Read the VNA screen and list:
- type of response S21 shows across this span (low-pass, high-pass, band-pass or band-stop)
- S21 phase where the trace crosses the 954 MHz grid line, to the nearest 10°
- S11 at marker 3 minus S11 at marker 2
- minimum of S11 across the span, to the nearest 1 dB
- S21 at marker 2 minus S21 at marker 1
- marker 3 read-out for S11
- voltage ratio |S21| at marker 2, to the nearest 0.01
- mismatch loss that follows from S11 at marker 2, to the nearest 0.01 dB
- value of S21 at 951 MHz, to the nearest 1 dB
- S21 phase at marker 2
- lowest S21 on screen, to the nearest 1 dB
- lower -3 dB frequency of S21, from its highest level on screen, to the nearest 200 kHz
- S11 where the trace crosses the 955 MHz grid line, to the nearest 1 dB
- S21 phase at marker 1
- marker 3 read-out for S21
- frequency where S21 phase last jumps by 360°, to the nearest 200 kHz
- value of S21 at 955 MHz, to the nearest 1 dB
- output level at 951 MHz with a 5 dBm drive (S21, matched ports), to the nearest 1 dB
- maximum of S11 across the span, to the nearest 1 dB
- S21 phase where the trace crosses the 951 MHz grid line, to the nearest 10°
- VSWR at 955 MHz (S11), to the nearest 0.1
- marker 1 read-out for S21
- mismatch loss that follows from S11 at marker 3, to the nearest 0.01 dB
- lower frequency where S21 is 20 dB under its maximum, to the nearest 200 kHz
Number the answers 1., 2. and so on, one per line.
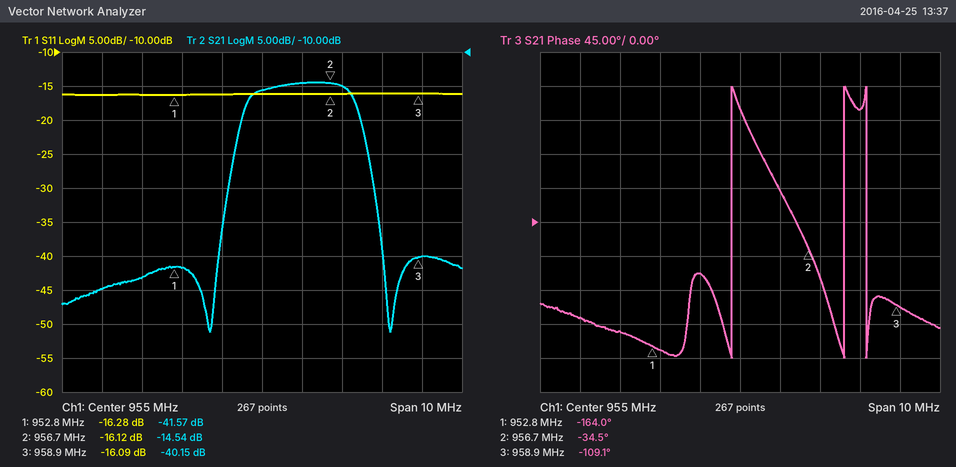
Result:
1. band-pass
2. -70°
3. 0.03 dB
4. -16 dB
5. 27.03 dB
6. -16.09 dB
7. 0.19
8. 0.11 dB
9. -45 dB
10. -34.5°
11. -51 dB
12. 954.6 MHz
13. -16 dB
14. -164.0°
15. -40.15 dB
16. 958.2 MHz
17. -16 dB
18. -40 dBm
19. -16 dB
20. -130°
21. 1.4
22. -41.57 dB
23. 0.11 dB
24. 954.0 MHz
